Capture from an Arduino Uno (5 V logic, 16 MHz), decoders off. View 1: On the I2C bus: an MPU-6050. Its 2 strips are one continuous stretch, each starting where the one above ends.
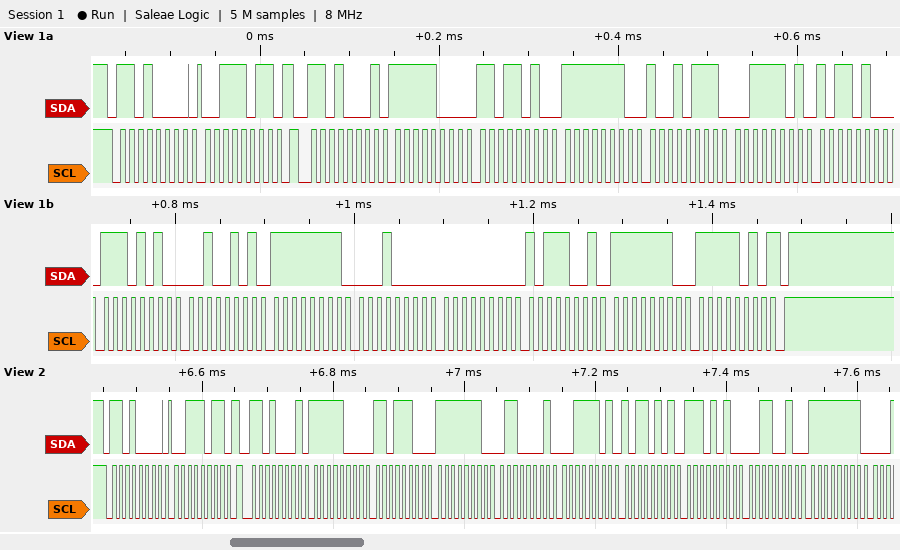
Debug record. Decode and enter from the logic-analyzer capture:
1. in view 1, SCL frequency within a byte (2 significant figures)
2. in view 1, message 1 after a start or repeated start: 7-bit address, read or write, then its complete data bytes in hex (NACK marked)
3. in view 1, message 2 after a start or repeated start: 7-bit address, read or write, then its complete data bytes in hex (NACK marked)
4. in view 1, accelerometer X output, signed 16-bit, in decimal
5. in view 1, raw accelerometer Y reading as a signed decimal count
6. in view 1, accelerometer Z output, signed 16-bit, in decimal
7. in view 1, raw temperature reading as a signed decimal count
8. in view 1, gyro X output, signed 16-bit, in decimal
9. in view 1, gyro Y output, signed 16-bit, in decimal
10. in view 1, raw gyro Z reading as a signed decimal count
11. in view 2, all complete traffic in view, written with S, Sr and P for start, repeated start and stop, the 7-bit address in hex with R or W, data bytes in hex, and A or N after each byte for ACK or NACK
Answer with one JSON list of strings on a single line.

["100 kHz", "0x68 write: 3B", "0x68 read: F8 DA FE 97 3D B4 EA 25 FF 10 00 B9 FE FA NACK", "-1830", "-361", "15796", "-5595", "-240", "185", "-262", "S 68W A 3B A Sr 68R A F8 A DC A FE A 61 A 3D A B5 A EA A 32 A FF A"]
